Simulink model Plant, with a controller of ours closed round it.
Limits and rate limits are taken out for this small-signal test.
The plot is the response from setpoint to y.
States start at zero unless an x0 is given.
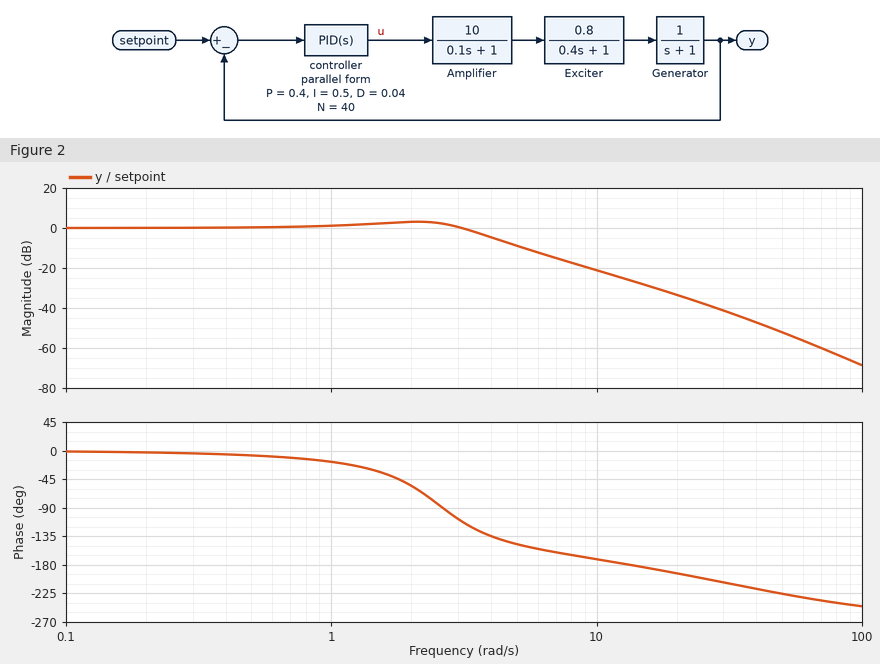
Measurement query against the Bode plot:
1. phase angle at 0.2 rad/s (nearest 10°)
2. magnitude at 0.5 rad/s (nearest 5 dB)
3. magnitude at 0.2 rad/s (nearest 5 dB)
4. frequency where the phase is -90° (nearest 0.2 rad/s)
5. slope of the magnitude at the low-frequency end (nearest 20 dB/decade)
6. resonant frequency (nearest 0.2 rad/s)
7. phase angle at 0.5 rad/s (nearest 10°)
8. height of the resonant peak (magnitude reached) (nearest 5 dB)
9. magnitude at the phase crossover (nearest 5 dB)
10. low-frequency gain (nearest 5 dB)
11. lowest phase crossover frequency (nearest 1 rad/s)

0°
0 dB
0 dB
2.6 rad/s
0 dB/decade
2.0 rad/s
-10°
5 dB
-25 dB
0 dB
13 rad/s
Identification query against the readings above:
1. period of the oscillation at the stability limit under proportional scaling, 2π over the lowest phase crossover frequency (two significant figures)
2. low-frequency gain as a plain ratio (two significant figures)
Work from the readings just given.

0.48 s
1.0
